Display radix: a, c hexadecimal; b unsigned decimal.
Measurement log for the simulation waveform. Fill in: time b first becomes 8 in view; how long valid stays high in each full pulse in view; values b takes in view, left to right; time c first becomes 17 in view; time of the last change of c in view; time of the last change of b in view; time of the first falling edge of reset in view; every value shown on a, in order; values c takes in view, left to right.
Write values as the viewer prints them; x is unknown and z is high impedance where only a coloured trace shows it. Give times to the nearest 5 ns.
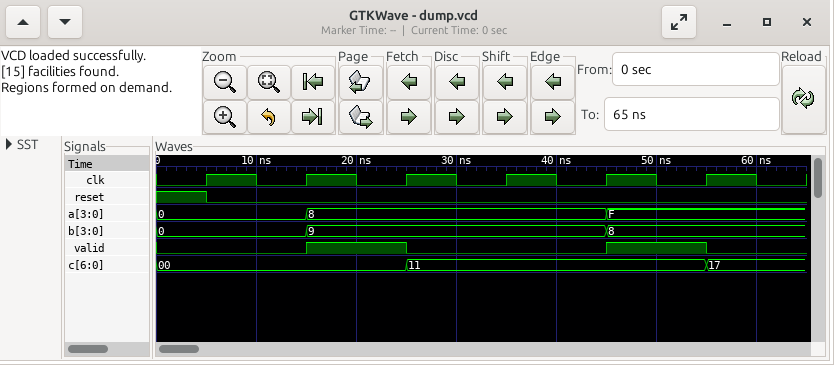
45 ns
10 ns, 10 ns
0, 9, 8
55 ns
55 ns
45 ns
5 ns
0, 8, F
00, 11, 17
